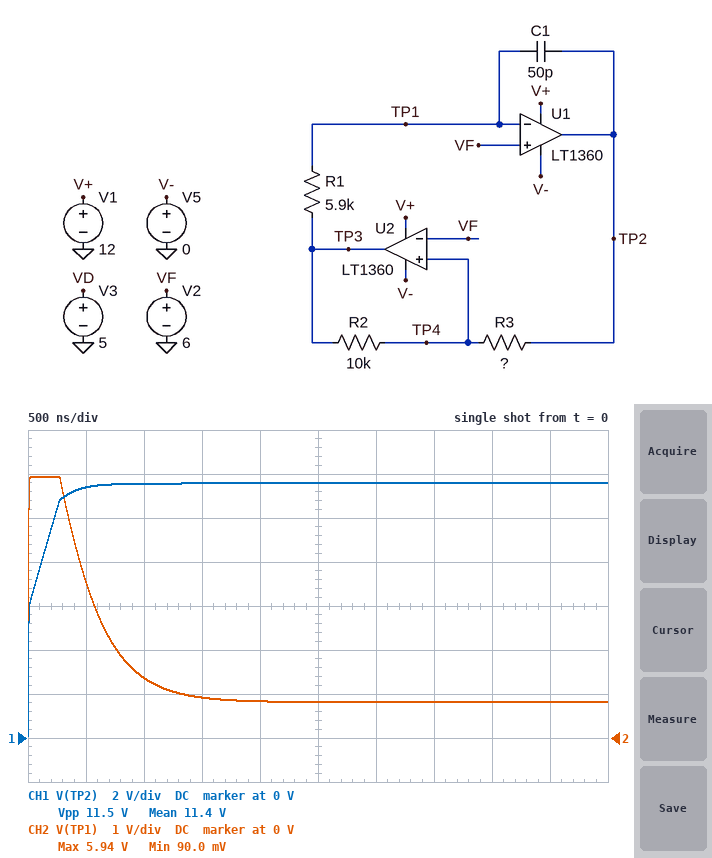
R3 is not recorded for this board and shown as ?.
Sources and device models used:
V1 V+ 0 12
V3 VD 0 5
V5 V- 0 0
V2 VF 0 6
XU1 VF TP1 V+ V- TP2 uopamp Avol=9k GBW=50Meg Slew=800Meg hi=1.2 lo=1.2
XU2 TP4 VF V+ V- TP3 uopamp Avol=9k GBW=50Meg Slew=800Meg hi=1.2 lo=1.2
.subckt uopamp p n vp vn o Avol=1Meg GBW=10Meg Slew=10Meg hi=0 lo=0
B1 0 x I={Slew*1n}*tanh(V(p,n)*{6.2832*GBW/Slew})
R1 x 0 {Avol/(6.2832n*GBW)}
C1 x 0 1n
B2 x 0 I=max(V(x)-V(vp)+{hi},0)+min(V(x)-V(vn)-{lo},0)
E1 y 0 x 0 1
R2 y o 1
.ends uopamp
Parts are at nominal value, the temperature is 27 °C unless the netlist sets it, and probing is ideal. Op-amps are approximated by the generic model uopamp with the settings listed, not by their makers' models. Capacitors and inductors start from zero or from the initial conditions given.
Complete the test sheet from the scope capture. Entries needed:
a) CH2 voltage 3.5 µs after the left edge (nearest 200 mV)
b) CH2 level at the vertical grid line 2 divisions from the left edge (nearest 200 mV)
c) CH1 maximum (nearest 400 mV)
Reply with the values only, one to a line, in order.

800 mV
1.4 V
11.6 V
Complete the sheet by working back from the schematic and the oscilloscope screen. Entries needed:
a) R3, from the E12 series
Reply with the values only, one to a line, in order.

18 kΩ
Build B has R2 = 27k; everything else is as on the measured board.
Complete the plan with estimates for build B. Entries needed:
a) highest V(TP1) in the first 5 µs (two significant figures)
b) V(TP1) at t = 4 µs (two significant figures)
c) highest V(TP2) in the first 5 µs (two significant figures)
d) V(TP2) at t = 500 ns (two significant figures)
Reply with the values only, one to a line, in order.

6.1 V
5.9 V
9.6 V
4.7 V
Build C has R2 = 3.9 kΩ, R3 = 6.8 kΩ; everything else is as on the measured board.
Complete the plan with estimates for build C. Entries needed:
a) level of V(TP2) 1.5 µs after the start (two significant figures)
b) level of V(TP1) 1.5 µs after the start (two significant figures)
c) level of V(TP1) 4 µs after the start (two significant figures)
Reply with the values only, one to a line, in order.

12 V
940 mV
840 mV
